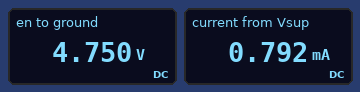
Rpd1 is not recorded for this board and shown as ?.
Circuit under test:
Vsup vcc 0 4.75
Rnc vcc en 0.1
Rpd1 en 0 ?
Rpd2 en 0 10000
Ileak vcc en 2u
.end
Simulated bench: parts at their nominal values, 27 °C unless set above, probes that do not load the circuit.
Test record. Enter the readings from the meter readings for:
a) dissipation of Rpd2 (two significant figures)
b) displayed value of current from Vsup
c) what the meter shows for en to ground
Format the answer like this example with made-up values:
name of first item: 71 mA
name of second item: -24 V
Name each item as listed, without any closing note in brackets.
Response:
dissipation of Rpd2: 2.3 mW
displayed value of current from Vsup: 0.792 mA
what the meter shows for en to ground: 4.750 V
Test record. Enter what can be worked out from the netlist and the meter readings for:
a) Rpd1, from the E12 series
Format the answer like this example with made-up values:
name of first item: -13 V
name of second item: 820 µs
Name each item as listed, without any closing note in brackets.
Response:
Rpd1, from the E12 series: 15 kΩ
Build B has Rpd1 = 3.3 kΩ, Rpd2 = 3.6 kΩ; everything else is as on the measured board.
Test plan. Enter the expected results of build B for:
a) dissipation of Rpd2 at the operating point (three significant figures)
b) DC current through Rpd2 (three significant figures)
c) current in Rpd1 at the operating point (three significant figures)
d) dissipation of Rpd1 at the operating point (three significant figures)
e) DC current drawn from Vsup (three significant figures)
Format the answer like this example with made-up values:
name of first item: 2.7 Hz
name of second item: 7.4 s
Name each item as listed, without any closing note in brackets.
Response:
dissipation of Rpd2 at the operating point: 6.27 mW
DC current through Rpd2: 1.32 mA
current in Rpd1 at the operating point: 1.44 mA
dissipation of Rpd1 at the operating point: 6.84 mW
DC current drawn from Vsup: 2.76 mA
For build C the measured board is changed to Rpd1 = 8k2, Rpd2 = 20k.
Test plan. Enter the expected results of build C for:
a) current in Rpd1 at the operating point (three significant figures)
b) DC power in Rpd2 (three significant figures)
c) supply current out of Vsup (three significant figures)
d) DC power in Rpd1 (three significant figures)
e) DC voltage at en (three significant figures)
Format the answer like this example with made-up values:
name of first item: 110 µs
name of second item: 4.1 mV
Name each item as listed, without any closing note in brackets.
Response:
current in Rpd1 at the operating point: 579 µA
DC power in Rpd2: 1.13 mW
supply current out of Vsup: 817 µA
DC power in Rpd1: 2.75 mW
DC voltage at en: 4.75 V
